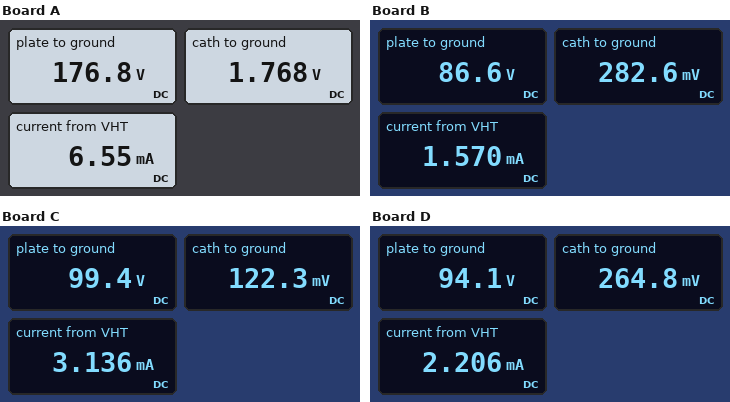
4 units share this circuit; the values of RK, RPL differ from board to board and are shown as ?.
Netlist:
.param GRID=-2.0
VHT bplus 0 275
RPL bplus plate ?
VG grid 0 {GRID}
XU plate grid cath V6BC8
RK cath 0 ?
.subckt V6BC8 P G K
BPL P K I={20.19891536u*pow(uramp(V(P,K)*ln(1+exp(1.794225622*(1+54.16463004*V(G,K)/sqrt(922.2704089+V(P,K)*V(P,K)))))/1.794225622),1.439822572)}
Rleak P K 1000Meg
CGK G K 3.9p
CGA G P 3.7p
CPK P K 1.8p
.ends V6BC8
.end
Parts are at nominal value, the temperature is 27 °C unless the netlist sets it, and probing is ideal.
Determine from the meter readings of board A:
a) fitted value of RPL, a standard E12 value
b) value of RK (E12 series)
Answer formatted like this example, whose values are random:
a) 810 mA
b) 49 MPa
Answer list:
a) 15 kΩ
b) 270 Ω
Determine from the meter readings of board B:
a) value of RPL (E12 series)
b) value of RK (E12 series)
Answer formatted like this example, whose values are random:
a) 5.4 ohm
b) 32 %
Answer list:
a) 120 kΩ
b) 180 Ω
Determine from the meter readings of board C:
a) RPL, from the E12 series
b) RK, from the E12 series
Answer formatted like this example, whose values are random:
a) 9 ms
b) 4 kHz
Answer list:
a) 56 kΩ
b) 39 Ω
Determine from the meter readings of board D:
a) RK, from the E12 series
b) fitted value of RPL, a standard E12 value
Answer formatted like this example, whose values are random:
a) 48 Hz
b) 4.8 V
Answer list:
a) 120 Ω
b) 82 kΩ
